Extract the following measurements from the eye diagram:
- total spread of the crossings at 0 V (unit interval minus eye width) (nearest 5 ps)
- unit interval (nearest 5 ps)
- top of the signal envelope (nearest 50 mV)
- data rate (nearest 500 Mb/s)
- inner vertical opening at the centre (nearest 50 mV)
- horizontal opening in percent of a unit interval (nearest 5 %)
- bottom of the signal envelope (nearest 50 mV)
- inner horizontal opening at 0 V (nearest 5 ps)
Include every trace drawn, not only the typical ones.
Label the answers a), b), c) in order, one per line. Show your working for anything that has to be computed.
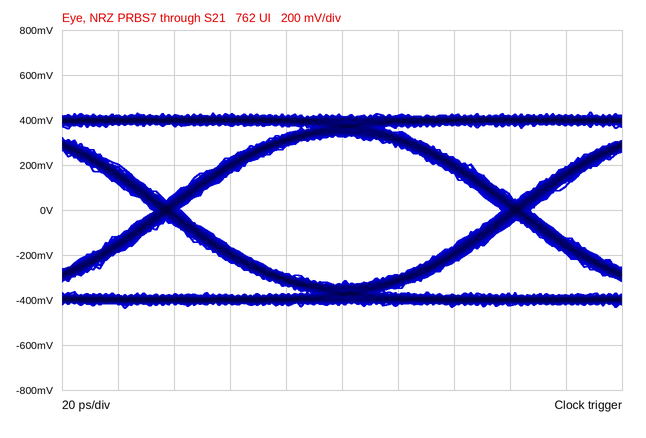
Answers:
a) 10 ps
b) 125 ps
c) 450 mV
d) 8.0 Gb/s
e) 650 mV
f) 115 ps / 125 ps ≈ 92.0 %, so 90 % to the nearest 5 %
g) -450 mV
h) 115 ps
